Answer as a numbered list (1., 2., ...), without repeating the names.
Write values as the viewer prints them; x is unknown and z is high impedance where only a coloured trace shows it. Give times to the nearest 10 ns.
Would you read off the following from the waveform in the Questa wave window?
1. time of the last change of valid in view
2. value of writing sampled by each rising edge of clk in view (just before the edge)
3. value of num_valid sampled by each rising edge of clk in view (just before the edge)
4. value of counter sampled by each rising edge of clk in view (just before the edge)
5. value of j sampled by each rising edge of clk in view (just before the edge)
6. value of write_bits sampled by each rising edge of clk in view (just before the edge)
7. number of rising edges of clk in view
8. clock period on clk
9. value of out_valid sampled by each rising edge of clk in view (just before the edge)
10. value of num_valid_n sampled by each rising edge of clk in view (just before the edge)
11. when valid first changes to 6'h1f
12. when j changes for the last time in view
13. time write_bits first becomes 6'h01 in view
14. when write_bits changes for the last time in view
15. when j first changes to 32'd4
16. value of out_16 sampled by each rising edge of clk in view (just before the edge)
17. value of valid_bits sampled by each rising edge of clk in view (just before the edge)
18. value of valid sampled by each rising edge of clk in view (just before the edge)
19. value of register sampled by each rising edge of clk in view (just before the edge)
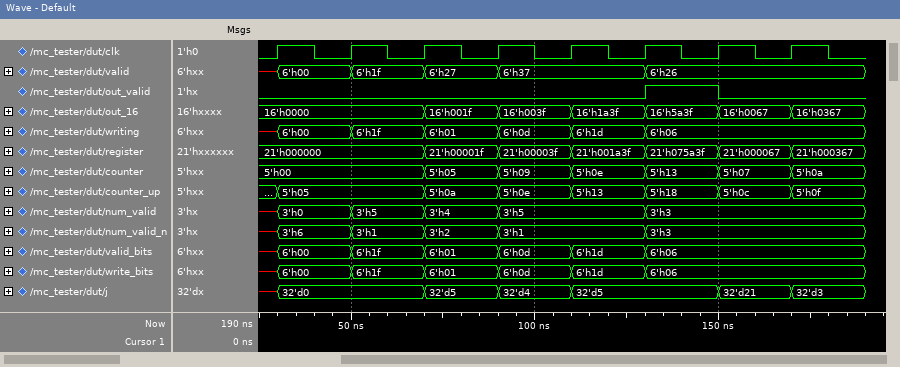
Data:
1. 130 ns
2. x, 6'h00, 6'h1f, 6'h01, 6'h0d, 6'h1d, 6'h06, 6'h06
3. x, 3'h0, 3'h5, 3'h4, 3'h5, 3'h5, 3'h3, 3'h3
4. 5'h00, 5'h00, 5'h00, 5'h05, 5'h09, 5'h0e, 5'h13, 5'h07
5. x, 32'd0, 32'd0, 32'd5, 32'd4, 32'd5, 32'd5, 32'd21
6. x, 6'h00, 6'h1f, 6'h01, 6'h0d, 6'h1d, 6'h06, 6'h06
7. 8
8. 20 ns
9. 0 0 0 0 0 0 1 0
10. x, 3'h6, 3'h1, 3'h2, 3'h1, 3'h1, 3'h3, 3'h3
11. 50 ns
12. 170 ns
13. 70 ns
14. 130 ns
15. 90 ns
16. 16'h0000, 16'h0000, 16'h0000, 16'h001f, 16'h003f, 16'h1a3f, 16'h5a3f, 16'h0067
17. x, 6'h00, 6'h1f, 6'h01, 6'h0d, 6'h1d, 6'h06, 6'h06
18. x, 6'h00, 6'h1f, 6'h27, 6'h37, 6'h37, 6'h26, 6'h26
19. 21'h000000, 21'h000000, 21'h000000, 21'h00001f, 21'h00003f, 21'h001a3f, 21'h075a3f, 21'h000067
